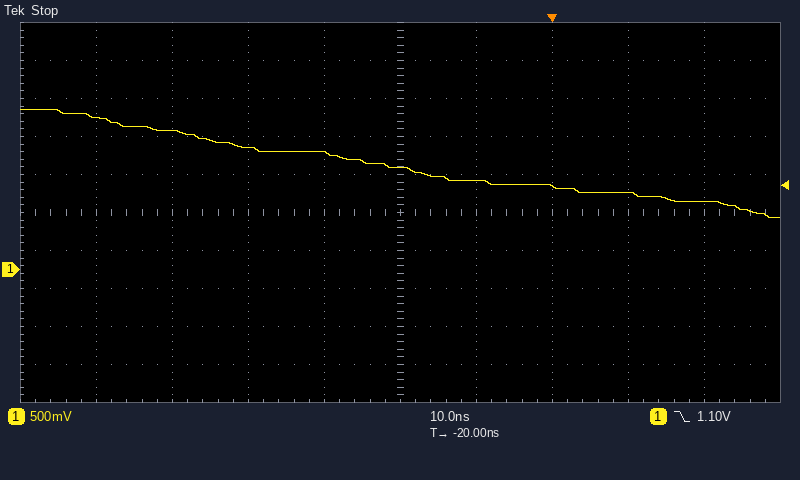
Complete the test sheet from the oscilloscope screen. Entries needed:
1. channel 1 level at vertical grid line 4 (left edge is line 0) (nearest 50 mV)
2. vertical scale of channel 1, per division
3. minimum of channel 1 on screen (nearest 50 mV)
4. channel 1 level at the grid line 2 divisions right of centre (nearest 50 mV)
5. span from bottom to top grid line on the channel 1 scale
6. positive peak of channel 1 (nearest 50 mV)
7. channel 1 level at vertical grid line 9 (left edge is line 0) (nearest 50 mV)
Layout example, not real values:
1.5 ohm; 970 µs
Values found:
1.55 V; 500 mV; 700 mV; 1.10 V; 5 V; 2.10 V; 900 mV
